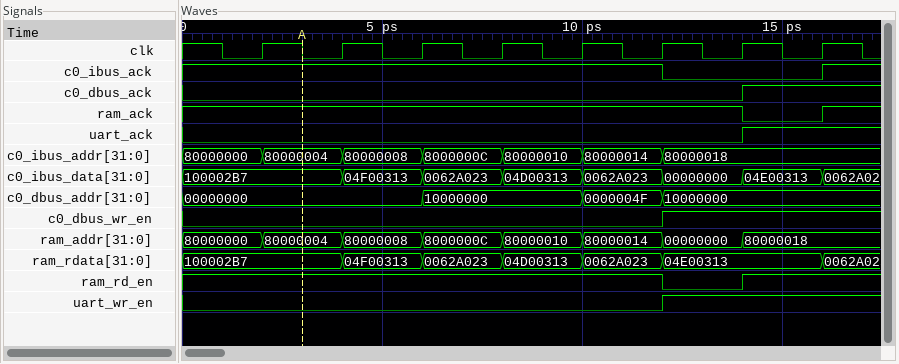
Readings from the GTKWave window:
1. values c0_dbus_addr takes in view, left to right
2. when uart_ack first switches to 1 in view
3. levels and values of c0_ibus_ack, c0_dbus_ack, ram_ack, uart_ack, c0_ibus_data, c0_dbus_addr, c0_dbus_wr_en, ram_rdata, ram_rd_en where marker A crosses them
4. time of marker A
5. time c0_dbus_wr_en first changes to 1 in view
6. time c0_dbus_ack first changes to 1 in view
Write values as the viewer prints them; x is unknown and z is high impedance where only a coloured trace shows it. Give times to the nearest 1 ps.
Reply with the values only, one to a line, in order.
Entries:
00000000, 10000000, 0000004F, 10000000
14 ps
c0_ibus_ack=1, c0_dbus_ack=0, ram_ack=1, uart_ack=0, c0_ibus_data=100002B7, c0_dbus_addr=00000000, c0_dbus_wr_en=0, ram_rdata=100002B7, ram_rd_en=1
3 ps
12 ps
14 ps
